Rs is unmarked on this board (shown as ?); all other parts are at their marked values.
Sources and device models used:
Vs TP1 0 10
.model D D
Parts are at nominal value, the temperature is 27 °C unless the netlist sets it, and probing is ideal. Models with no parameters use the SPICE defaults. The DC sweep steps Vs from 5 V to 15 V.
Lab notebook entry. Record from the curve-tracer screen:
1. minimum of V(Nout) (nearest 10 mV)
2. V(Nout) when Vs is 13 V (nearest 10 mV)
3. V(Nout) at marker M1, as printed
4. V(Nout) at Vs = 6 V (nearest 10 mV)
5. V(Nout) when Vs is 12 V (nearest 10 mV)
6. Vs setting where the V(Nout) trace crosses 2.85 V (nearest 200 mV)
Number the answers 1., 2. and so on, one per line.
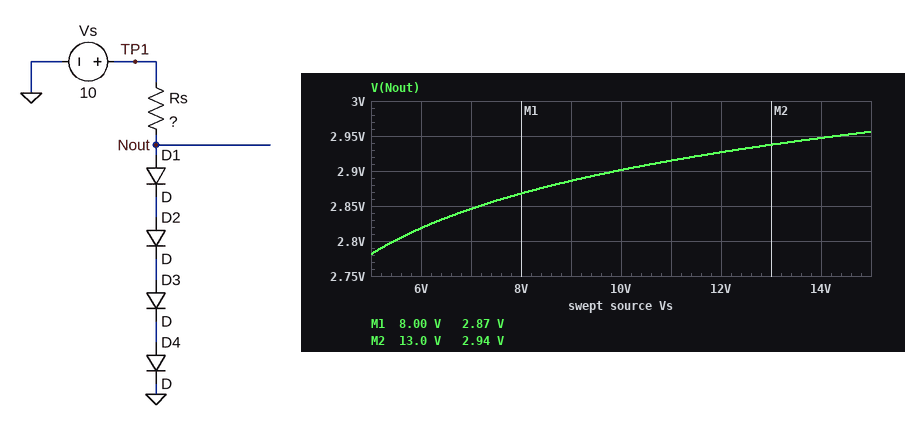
1. 2.78 V
2. 2.94 V
3. 2.87 V
4. 2.82 V
5. 2.93 V
6. 7.2 V
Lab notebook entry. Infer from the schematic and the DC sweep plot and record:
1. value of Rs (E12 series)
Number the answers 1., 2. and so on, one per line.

1. 470 Ω
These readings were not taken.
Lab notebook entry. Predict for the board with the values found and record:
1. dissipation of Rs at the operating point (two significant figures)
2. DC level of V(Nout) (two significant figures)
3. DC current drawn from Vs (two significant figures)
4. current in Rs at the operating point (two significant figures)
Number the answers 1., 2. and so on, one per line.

1. 110 mW
2. 2.9 V
3. 15 mA
4. 15 mA
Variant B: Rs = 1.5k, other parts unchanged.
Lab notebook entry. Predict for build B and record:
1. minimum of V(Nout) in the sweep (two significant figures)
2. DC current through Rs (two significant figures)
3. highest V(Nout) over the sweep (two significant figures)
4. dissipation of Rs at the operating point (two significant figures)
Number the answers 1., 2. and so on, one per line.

1. 2.7 V
2. 4.8 mA
3. 2.8 V
4. 35 mW
